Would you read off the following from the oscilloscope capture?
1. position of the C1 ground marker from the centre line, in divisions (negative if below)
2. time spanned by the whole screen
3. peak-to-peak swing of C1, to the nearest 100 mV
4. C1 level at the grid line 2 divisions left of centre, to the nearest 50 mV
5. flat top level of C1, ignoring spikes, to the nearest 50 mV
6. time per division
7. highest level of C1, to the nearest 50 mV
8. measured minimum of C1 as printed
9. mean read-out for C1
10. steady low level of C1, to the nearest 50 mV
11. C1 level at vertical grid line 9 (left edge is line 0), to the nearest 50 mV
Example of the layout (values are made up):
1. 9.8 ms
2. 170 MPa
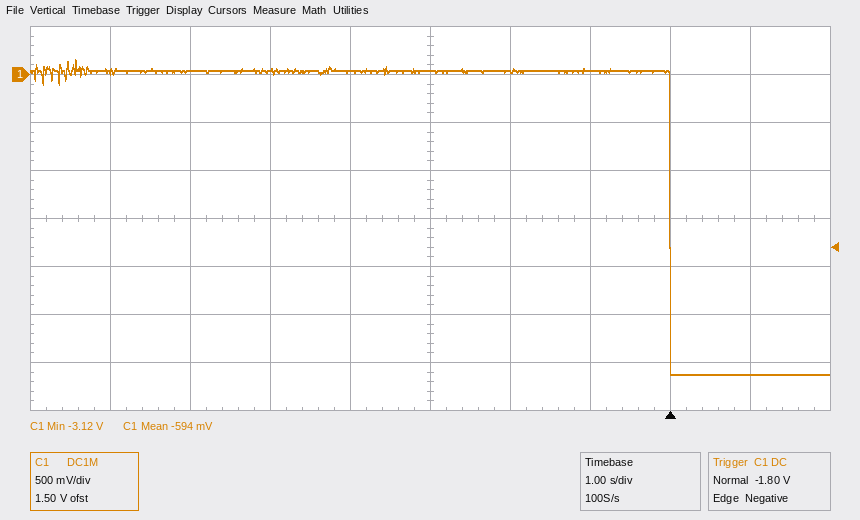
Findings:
1. +3.0 div
2. 10 s
3. 3.30 V
4. 50 mV
5. 50 mV
6. 1 s
7. 150 mV
8. -3.12 V
9. -594 mV
10. -3.10 V
11. -3.10 V
